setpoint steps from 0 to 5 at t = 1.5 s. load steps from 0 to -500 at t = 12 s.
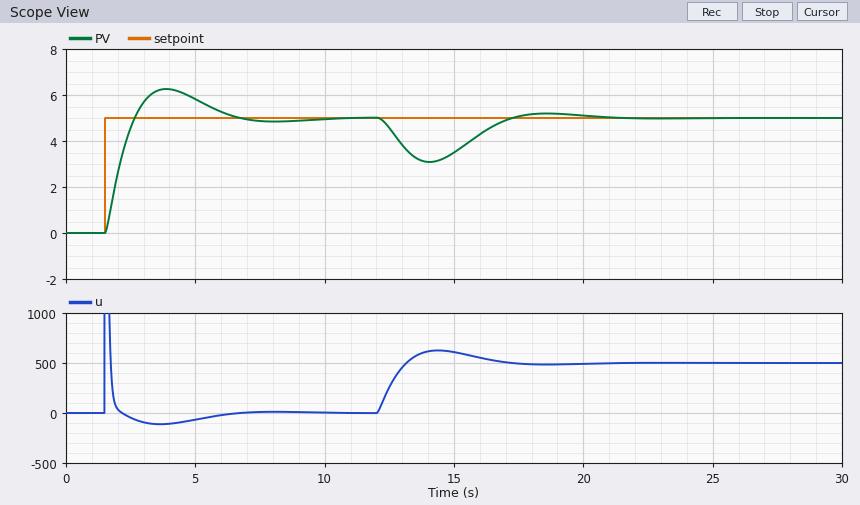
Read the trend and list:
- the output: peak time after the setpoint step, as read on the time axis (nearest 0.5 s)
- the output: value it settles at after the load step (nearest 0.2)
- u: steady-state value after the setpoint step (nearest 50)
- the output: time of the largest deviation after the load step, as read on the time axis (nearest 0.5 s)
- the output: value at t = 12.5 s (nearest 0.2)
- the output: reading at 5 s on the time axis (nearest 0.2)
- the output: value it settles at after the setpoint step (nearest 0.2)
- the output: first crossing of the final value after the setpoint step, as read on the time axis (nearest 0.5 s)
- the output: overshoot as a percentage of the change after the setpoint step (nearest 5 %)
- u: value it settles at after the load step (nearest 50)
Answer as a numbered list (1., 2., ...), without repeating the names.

1. 4.0 s
2. 5.0
3. 0
4. 14.0 s
5. 4.6
6. 5.8
7. 5.0
8. 2.5 s
9. 25 %
10. 500
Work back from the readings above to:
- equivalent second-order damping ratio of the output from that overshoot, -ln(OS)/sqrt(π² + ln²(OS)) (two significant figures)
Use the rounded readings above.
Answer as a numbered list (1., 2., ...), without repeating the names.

1. 0.40
